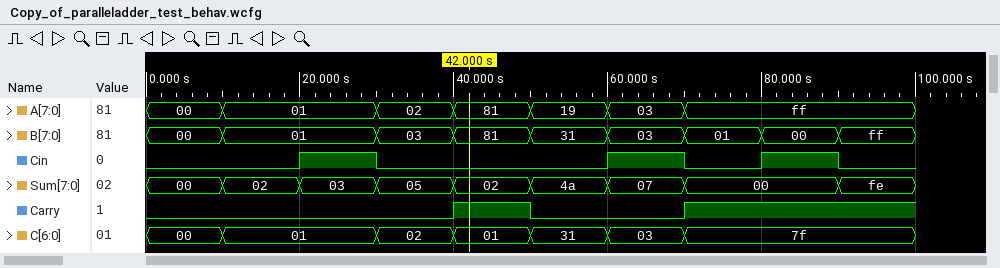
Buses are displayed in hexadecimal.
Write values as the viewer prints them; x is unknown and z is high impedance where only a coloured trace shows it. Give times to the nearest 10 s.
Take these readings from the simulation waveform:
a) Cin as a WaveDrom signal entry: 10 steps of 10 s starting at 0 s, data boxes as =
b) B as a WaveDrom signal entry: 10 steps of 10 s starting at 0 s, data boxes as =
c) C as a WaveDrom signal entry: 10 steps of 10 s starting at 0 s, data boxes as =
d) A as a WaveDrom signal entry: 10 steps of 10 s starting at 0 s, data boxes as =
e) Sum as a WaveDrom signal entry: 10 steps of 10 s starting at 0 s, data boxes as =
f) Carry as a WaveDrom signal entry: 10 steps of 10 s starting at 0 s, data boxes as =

{name: 'Cin', wave: '0.10..1010'}
{name: 'B', wave: '==.=======', data: '00 01 03 81 31 03 01 00 ff'}
{name: 'C', wave: '==.=====..', data: '00 01 02 01 31 03 7f'}
{name: 'A', wave: '==.=====..', data: '00 01 02 81 19 03 ff'}
{name: 'Sum', wave: '========.=', data: '00 02 03 05 02 4a 07 00 fe'}
{name: 'Carry', wave: '0...10.1..'}
